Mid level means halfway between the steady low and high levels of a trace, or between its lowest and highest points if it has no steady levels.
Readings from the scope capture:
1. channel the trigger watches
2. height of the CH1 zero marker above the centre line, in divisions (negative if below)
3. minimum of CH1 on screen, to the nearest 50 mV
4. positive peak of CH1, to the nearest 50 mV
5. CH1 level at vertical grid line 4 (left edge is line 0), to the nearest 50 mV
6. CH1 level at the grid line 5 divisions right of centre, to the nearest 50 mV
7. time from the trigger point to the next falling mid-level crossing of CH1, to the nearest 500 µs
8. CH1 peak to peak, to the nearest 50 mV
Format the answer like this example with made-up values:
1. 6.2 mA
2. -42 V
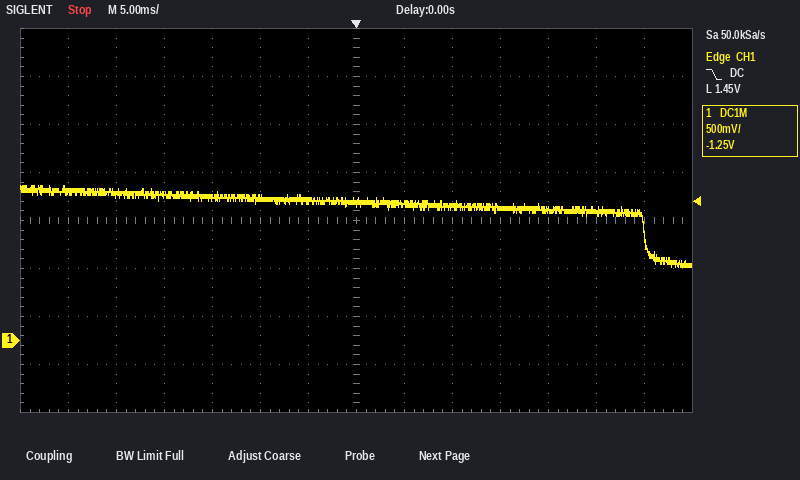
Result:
1. CH1
2. -2.5 div
3. 750 mV
4. 1.60 V
5. 1.50 V
6. 1.35 V
7. 30.0 ms
8. 850 mV
